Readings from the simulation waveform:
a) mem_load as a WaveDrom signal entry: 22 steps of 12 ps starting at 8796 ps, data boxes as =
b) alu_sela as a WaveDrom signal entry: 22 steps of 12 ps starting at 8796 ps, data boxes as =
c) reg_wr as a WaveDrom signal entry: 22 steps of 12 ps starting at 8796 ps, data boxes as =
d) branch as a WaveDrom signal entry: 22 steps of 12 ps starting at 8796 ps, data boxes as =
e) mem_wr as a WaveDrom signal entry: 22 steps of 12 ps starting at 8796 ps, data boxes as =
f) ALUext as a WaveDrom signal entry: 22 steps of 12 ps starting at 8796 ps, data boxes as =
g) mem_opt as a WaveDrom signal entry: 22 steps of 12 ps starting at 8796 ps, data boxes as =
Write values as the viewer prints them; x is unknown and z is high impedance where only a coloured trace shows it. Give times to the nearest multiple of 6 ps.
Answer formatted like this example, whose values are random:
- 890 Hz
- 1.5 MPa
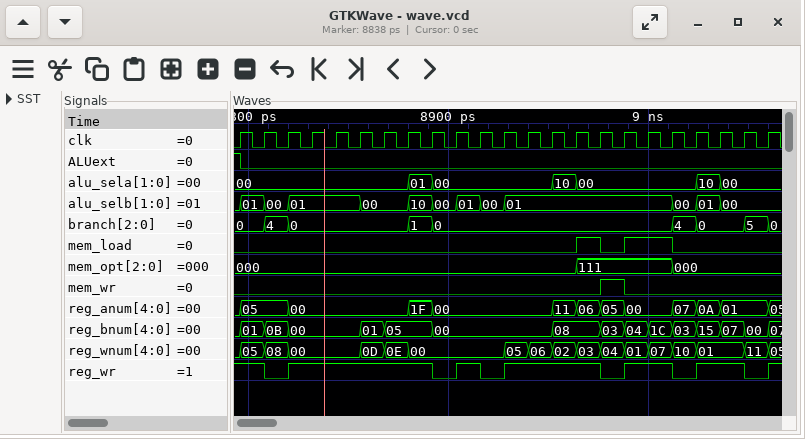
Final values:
- {name: 'mem_load', wave: '0.............101.0...'}
- {name: 'alu_sela', wave: '=......==....==....==.', data: '00 01 00 10 00 10 00'}
- {name: 'reg_wr', wave: '101.....0101...01.01.0'}
- {name: 'branch', wave: '===....==.........==.=', data: '0 4 0 1 0 4 0 5'}
- {name: 'mem_wr', wave: '0..............10.....'}
- {name: 'ALUext', wave: '0.....................'}
- {name: 'mem_opt', wave: '=.............=...=...', data: '000 111 000'}
